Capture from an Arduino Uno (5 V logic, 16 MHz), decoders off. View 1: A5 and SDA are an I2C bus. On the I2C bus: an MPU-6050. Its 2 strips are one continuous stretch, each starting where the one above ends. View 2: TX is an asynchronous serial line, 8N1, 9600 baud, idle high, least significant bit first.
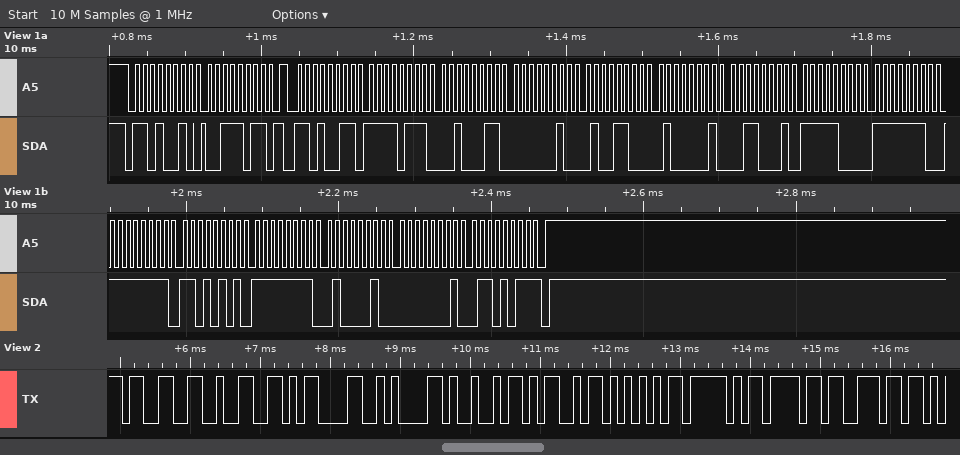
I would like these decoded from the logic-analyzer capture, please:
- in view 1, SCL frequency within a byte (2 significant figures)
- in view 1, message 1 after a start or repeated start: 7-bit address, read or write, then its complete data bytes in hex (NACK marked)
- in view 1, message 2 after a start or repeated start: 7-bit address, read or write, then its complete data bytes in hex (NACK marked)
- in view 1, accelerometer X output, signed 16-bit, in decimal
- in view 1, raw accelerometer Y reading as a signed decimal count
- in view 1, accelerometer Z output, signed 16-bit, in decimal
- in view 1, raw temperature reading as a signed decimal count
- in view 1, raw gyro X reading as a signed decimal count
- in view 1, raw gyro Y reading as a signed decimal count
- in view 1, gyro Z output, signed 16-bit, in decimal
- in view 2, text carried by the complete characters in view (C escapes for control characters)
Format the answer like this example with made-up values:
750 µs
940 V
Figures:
100 kHz
0x69 write: 3B
0x69 read: F7 23 02 4C 41 31 F8 FE FF D5 FF 42 01 6B NACK
-2269
588
16689
-1794
-43
-190
363
"32\r\nIMU_on"
